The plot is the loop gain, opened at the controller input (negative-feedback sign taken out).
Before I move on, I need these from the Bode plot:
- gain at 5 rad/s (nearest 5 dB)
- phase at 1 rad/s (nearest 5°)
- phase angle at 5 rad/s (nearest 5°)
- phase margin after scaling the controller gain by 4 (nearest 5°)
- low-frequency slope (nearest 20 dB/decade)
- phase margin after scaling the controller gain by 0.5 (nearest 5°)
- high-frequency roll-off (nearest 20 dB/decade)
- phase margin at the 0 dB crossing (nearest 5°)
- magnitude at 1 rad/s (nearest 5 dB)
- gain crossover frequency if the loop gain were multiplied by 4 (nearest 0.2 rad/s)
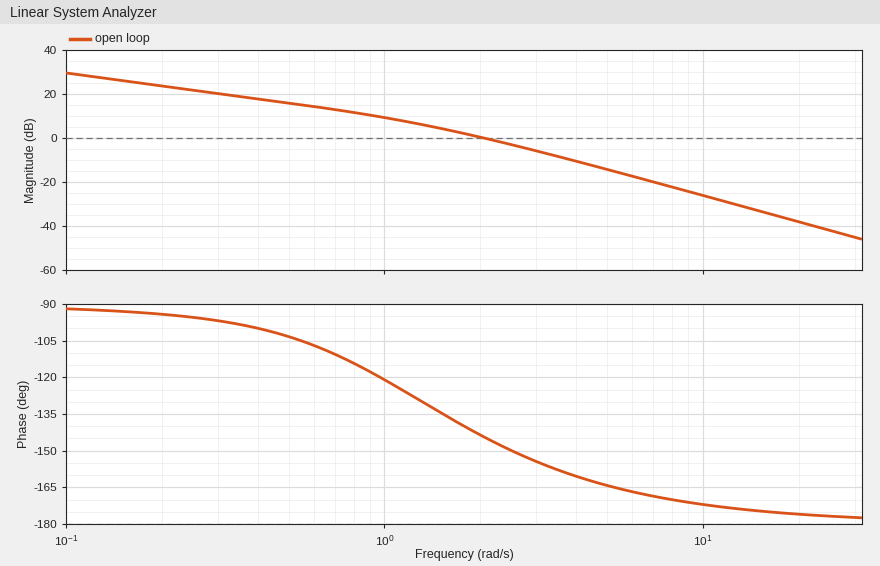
-15 dB
-120°
-165°
20°
-20 dB/decade
50°
-40 dB/decade
35°
10 dB
4.4 rad/s
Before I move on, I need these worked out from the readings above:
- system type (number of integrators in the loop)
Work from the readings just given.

1
